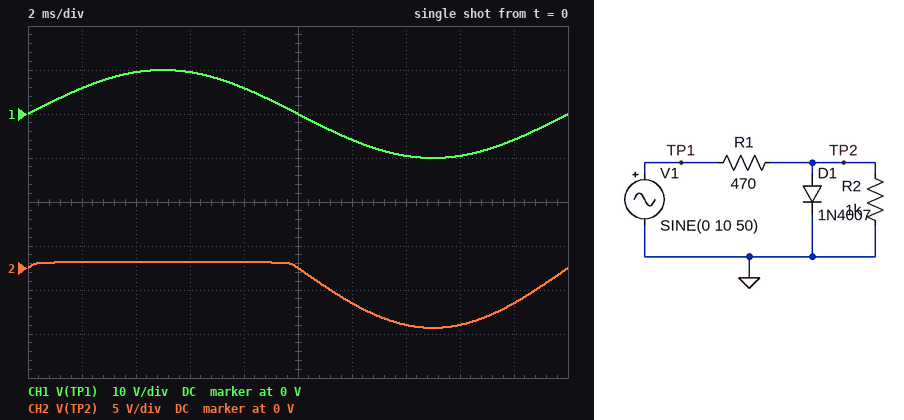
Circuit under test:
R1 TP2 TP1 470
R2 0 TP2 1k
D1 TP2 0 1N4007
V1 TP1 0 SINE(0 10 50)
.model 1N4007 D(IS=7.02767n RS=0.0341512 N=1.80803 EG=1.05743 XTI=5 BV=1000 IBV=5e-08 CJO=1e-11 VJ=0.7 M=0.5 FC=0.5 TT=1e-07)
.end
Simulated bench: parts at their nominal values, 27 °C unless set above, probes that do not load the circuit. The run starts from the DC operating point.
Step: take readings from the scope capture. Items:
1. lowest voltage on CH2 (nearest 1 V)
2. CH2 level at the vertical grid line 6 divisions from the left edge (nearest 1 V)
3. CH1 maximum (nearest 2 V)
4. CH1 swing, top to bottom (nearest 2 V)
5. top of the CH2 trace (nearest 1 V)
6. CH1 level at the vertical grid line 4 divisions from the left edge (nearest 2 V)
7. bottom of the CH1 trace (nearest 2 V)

-7 V
-4 V
10 V
20 V
1 V
6 V
-10 V
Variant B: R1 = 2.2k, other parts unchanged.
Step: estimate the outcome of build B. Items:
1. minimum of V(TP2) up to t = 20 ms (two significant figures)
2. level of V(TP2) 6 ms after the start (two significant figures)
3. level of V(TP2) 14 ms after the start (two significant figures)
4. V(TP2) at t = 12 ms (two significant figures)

-3.1 V
610 mV
-3.0 V
-1.8 V
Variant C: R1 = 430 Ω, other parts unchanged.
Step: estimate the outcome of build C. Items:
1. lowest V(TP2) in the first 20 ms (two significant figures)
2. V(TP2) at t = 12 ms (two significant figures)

-7.0 V
-4.1 V
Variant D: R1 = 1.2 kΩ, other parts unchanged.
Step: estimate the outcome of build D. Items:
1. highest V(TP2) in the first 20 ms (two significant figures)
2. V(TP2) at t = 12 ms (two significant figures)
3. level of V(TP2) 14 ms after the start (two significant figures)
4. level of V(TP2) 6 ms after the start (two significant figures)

650 mV
-2.7 V
-4.3 V
640 mV
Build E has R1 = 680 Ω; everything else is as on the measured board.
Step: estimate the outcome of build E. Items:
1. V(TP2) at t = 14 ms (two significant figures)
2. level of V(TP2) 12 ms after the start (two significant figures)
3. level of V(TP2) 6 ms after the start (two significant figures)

-5.7 V
-3.5 V
670 mV
